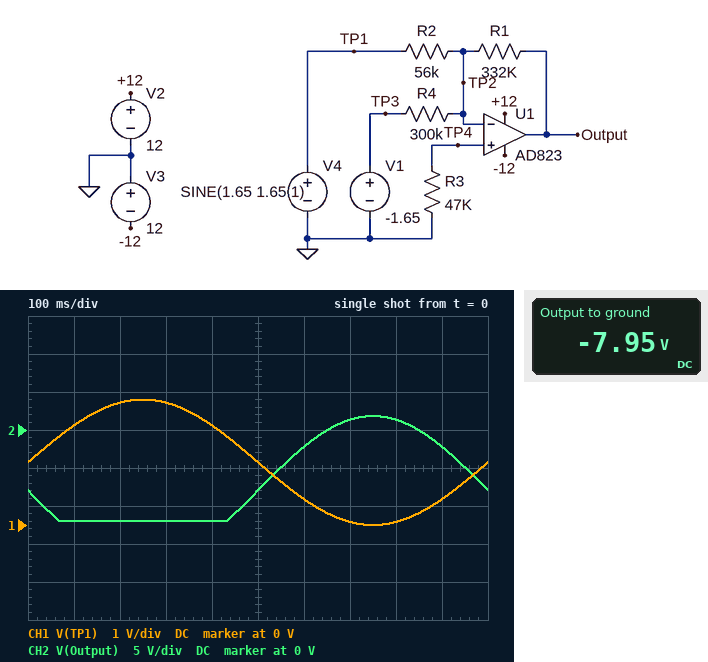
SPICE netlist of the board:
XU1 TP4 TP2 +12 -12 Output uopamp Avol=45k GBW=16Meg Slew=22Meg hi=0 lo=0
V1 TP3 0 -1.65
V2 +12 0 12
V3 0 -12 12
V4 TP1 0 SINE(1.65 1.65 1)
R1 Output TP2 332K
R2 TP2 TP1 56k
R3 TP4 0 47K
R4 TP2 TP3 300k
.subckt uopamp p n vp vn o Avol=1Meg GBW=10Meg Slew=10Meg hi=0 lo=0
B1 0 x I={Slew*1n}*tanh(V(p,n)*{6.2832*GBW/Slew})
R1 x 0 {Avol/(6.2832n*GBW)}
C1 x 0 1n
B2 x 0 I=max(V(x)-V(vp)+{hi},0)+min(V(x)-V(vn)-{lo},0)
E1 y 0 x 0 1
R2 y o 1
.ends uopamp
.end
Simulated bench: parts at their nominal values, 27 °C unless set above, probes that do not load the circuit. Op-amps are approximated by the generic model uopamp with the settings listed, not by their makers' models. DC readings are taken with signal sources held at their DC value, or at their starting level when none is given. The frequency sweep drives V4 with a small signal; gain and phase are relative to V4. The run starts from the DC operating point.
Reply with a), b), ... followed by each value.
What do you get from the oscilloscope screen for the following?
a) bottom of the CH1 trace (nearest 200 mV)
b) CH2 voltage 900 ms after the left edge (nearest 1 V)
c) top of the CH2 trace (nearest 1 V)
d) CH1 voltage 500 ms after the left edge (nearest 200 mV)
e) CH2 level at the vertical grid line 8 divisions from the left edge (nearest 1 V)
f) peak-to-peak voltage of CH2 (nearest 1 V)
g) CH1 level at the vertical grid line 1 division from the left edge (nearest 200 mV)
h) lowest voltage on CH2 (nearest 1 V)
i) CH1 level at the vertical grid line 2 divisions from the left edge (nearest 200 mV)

a) 0 V
b) -2 V
c) 2 V
d) 1.6 V
e) 1 V
f) 14 V
g) 2.6 V
h) -12 V
i) 3.2 V
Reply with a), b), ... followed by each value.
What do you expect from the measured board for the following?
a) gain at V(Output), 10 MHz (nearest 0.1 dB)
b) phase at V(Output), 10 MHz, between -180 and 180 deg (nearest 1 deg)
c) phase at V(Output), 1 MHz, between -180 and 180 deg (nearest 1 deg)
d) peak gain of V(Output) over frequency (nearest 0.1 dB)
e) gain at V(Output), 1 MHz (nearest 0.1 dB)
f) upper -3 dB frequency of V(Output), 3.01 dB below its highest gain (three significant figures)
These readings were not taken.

a) 1.3 dB
b) 101 deg
c) 153 deg
d) 15.5 dB
e) 14.5 dB
f) 1.99 MHz
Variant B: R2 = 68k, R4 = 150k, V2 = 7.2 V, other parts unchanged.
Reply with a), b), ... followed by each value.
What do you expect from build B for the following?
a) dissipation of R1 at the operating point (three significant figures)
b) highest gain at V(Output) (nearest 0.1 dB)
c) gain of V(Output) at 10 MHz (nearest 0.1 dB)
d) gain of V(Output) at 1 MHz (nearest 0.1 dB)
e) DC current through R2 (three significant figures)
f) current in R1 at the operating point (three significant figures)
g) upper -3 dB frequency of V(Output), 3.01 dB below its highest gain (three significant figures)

a) 58.4 µW
b) 13.8 dB
c) -0.5 dB
d) 12.8 dB
e) 24.3 µA
f) 13.3 µA
g) 1.98 MHz
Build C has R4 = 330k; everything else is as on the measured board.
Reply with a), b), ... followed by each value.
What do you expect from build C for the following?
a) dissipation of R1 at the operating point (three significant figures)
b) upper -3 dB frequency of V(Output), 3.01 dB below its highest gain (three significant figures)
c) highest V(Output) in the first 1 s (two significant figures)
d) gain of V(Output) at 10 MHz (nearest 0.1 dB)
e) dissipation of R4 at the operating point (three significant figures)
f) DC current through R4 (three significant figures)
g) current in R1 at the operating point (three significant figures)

a) 199 µW
b) 2.02 MHz
c) 1.7 V
d) 1.4 dB
e) 8.25 µW
f) 5.00 µA
g) 24.5 µA
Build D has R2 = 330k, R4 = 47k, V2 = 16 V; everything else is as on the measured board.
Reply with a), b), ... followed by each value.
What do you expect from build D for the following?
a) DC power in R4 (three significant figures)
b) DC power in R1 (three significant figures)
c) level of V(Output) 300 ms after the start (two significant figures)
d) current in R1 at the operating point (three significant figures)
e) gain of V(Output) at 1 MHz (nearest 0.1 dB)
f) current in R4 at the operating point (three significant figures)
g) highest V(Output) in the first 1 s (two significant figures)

a) 57.9 µW
b) 301 µW
c) 8.4 V
d) 30.1 µA
e) -1.2 dB
f) 35.1 µA
g) 12 V
